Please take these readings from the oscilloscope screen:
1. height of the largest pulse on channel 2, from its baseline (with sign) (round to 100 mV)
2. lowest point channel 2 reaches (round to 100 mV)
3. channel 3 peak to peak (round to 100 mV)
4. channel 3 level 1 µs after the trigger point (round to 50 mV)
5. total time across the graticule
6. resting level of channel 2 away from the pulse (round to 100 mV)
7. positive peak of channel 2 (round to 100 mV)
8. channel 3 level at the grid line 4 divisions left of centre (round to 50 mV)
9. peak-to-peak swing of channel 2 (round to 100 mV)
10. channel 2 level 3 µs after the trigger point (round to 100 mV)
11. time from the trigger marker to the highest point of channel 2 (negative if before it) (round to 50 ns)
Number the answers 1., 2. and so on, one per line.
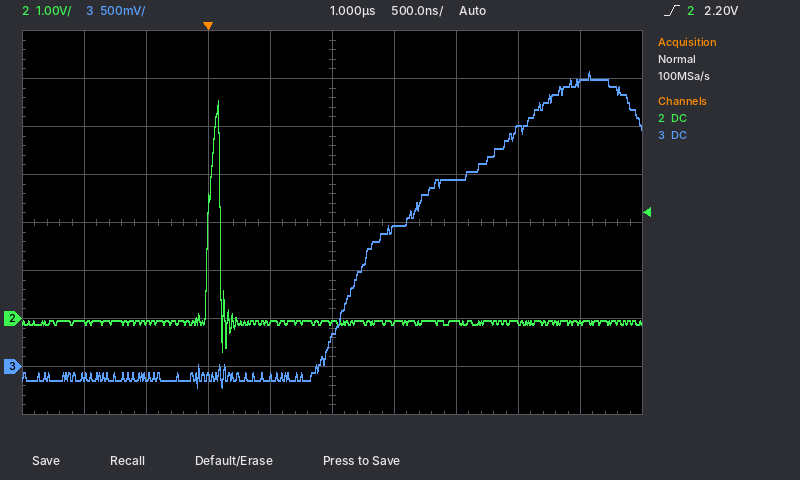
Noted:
1. +4.6 V
2. -700 mV
3. 3.30 V
4. 300 mV
5. 5 µs
6. -100 mV
7. 4.5 V
8. -100 mV
9. 5.2 V
10. -100 mV
11. +100 ns
